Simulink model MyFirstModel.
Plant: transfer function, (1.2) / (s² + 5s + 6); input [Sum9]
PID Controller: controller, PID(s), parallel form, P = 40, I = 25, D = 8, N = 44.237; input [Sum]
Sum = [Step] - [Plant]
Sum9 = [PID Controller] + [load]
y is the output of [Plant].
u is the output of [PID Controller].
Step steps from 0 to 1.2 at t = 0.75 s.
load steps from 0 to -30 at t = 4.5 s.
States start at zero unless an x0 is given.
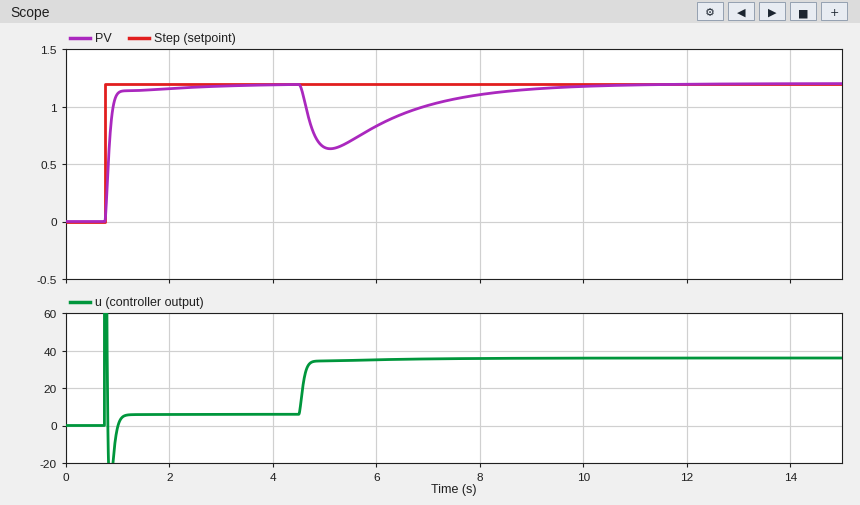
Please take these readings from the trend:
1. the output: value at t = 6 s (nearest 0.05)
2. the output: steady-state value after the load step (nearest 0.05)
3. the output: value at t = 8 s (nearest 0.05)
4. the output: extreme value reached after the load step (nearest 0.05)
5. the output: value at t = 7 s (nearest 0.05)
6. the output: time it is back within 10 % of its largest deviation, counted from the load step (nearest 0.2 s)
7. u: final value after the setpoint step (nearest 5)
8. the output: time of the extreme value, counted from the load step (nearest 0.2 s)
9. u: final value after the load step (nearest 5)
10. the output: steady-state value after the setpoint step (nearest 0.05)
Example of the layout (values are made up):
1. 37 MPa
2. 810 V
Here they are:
1. 0.85
2. 1.20
3. 1.10
4. 0.65
5. 1.00
6. 4.4 s
7. 5
8. 0.6 s
9. 35
10. 1.20
